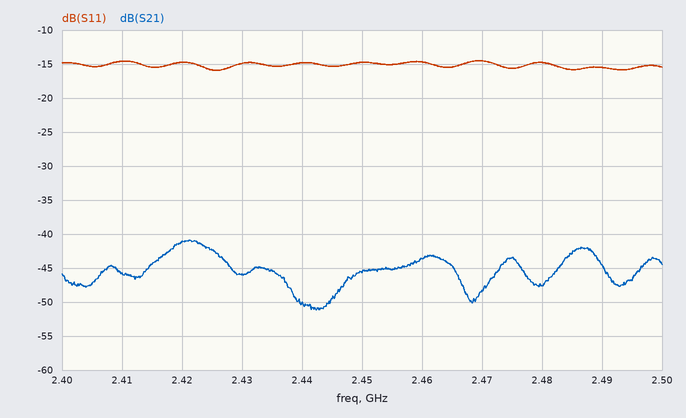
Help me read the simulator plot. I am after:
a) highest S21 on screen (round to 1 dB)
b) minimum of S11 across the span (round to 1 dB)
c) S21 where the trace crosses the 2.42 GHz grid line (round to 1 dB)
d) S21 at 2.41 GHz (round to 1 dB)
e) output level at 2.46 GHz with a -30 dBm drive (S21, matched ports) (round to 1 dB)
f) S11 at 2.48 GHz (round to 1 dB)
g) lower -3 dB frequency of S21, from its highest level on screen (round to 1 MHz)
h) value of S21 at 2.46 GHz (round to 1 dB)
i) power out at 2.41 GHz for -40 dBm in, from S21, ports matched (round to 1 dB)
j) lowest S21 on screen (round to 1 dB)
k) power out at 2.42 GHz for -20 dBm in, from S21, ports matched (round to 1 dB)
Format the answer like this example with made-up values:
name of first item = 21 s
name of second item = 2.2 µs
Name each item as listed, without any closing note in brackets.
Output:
highest S21 on screen = -41 dB
minimum of S11 across the span = -16 dB
S21 where the trace crosses the 2.42 GHz grid line = -41 dB
S21 at 2.41 GHz = -46 dB
output level at 2.46 GHz with a -30 dBm drive (S21, matched ports) = -74 dBm
S11 at 2.48 GHz = -15 dB
lower -3 dB frequency of S21, from its highest level on screen = 2.416 GHz
value of S21 at 2.46 GHz = -44 dB
power out at 2.41 GHz for -40 dBm in, from S21, ports matched = -86 dBm
lowest S21 on screen = -51 dB
power out at 2.42 GHz for -20 dBm in, from S21, ports matched = -61 dBm
